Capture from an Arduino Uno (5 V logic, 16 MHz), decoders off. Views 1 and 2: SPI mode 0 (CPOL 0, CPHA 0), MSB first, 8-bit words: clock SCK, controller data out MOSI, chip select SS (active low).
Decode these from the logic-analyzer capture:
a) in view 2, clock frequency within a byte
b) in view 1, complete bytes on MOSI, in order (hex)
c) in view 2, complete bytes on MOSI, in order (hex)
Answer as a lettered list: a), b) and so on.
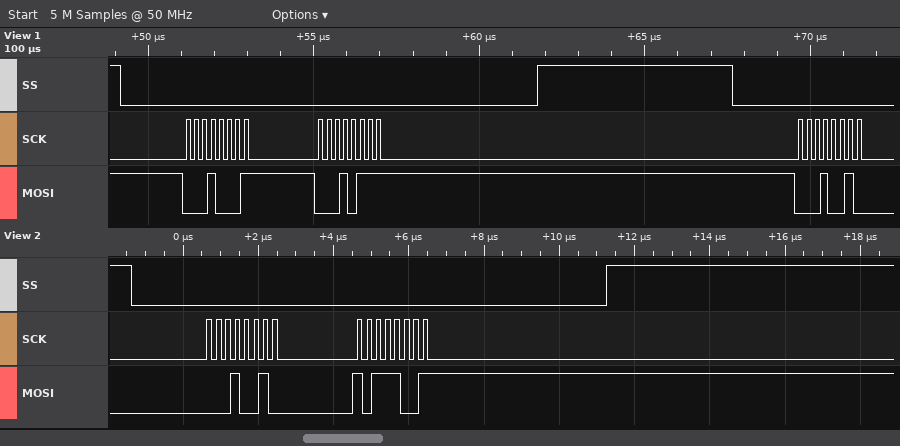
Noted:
a) 4 MHz
b) 11 17 12
c) 0x12 0xB9
